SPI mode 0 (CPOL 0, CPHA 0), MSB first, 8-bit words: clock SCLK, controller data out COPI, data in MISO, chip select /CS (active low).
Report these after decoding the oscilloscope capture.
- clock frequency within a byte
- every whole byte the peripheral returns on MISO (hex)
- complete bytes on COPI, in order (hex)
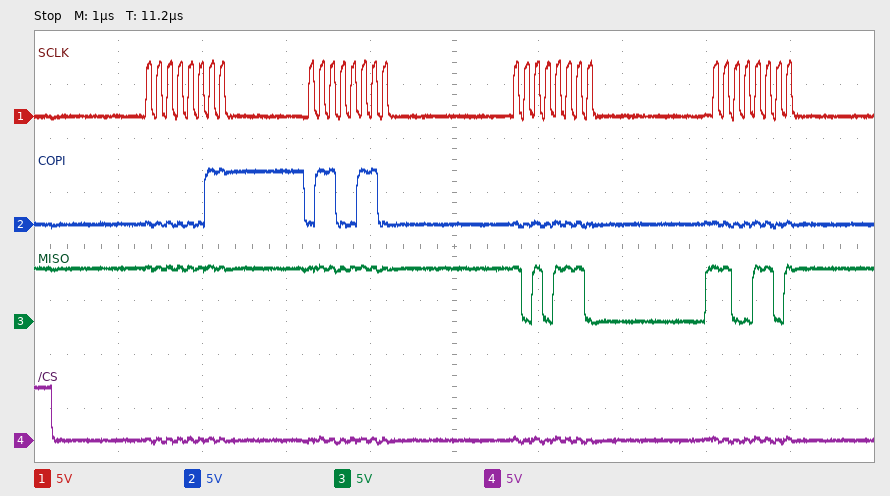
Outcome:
8 MHz
FF FF AE CD
03 66 00 00
